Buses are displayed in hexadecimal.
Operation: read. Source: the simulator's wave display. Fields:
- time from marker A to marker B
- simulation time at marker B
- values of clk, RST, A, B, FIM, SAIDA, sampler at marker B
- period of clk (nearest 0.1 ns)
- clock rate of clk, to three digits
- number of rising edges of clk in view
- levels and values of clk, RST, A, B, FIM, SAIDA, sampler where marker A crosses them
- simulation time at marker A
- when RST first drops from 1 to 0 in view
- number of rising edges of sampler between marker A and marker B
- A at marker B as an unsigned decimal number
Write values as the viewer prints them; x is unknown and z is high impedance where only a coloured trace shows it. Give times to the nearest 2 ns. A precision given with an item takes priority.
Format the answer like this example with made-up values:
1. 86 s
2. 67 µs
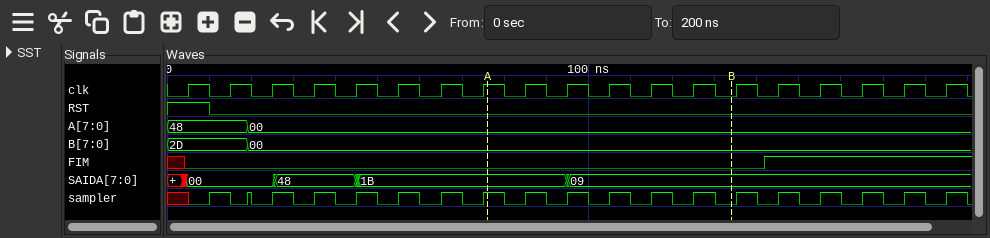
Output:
1. 58 ns
2. 134 ns
3. clk=0, RST=0, A=00, B=00, FIM=0, SAIDA=09, sampler=0
4. 10 ns
5. 100 MHz
6. 19
7. clk=1, RST=0, A=00, B=00, FIM=0, SAIDA=1B, sampler=1
8. 76 ns
9. 10 ns
10. 5
11. 0
